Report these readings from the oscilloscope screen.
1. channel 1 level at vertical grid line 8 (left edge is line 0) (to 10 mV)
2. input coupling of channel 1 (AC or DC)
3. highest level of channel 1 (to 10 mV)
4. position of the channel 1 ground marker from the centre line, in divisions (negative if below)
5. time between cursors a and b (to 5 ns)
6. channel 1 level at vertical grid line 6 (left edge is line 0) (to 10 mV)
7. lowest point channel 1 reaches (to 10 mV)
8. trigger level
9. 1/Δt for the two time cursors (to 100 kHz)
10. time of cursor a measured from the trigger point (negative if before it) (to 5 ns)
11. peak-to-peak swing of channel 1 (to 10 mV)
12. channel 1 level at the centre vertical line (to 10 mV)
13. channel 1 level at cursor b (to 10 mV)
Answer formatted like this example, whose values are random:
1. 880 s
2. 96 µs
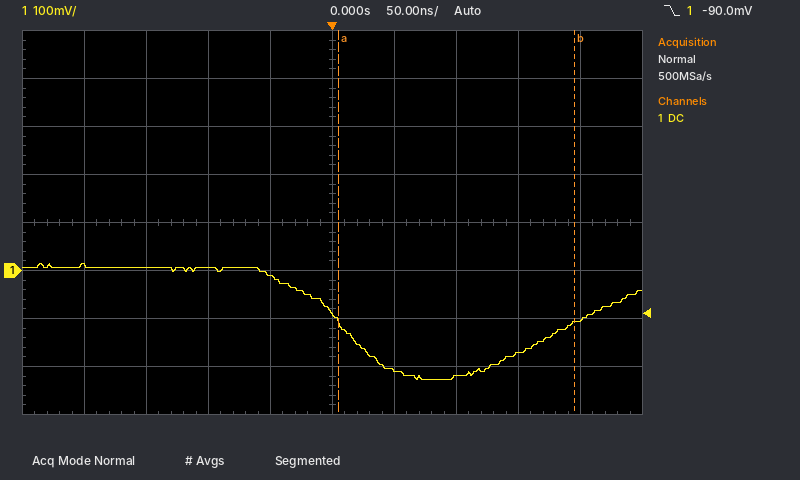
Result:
1. -170 mV
2. DC
3. 10 mV
4. -1.0 div
5. 190 ns
6. -210 mV
7. -230 mV
8. -90.0 mV
9. 5.3 MHz
10. +5 ns
11. 240 mV
12. -90 mV
13. -110 mV
